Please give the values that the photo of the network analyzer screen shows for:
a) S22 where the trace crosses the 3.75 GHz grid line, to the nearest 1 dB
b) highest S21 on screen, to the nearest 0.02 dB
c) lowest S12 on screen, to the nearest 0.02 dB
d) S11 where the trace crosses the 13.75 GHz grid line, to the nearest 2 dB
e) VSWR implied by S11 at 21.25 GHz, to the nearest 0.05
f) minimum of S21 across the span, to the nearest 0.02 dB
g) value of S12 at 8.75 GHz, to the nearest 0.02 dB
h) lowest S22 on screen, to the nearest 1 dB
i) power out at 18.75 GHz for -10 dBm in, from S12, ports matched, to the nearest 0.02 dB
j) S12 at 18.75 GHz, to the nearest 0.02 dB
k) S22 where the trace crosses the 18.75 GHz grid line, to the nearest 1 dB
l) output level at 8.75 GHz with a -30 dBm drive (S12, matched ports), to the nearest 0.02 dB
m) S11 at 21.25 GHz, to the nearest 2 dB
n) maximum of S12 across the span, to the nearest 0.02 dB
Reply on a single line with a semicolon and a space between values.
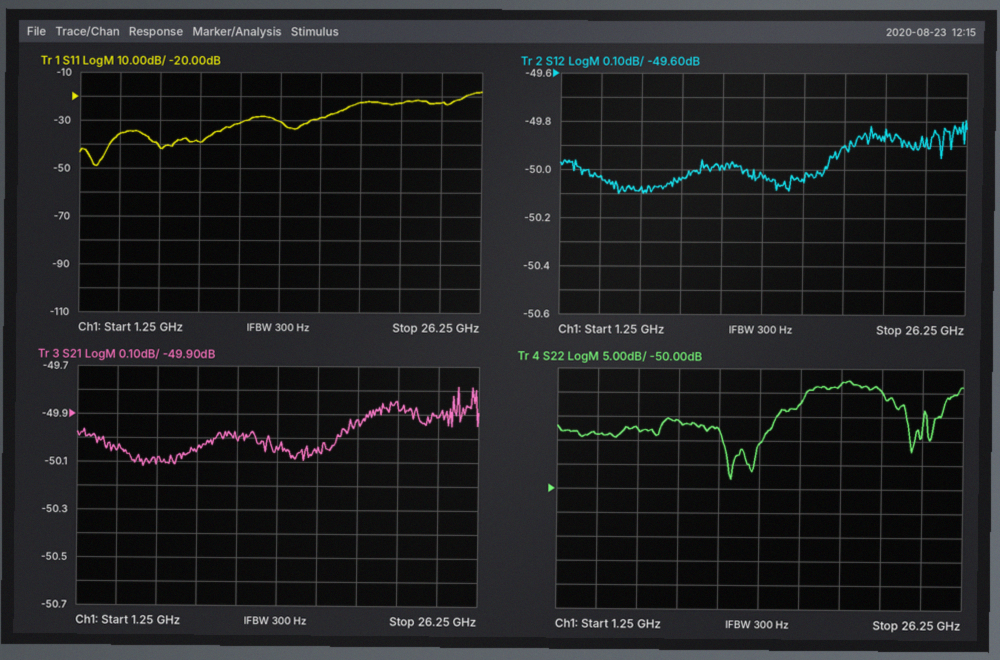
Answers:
-39 dB; -49.78 dB; -50.10 dB; -30 dB; 1.15; -50.12 dB; -50.04 dB; -48 dB; -59.90 dBm; -49.90 dB; -28 dB; -80.04 dBm; -22 dB; -49.80 dB
